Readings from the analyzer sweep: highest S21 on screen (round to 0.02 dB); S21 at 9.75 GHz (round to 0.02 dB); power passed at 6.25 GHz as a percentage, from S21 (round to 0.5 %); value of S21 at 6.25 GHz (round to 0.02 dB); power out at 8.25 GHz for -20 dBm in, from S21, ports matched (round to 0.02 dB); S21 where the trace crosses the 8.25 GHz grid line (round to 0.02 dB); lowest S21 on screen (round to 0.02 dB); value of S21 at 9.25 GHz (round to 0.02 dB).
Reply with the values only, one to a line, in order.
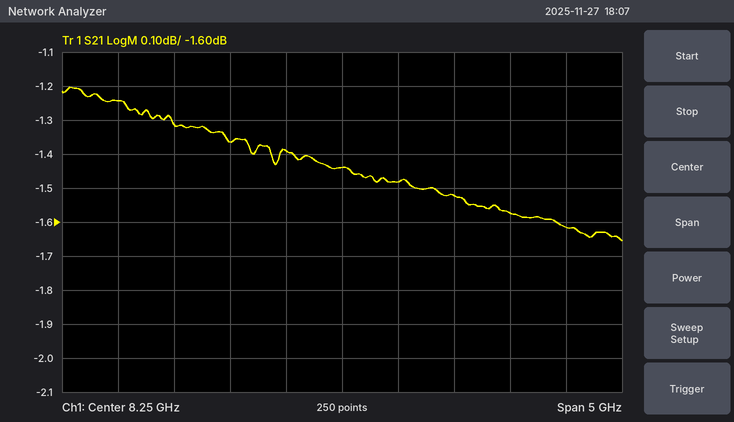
-1.20 dB
-1.58 dB
75.0 %
-1.24 dB
-21.44 dBm
-1.44 dB
-1.66 dB
-1.52 dB
